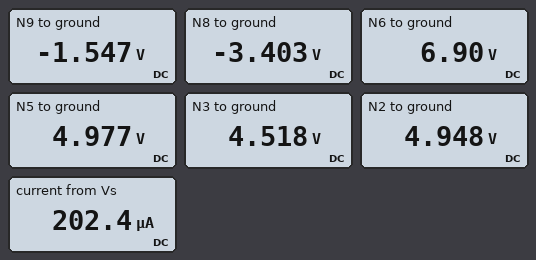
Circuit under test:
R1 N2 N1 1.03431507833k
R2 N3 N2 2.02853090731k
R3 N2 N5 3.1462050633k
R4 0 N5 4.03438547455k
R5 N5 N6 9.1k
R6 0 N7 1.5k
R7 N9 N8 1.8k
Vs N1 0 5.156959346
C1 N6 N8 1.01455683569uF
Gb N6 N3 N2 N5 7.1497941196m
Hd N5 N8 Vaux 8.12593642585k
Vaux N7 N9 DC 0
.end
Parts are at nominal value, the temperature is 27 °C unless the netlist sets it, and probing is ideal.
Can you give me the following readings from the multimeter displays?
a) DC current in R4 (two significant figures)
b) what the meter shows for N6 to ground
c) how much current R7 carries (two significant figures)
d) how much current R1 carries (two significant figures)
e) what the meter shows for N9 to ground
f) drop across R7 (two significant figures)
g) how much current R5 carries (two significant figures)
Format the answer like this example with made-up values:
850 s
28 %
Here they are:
1.2 mA
6.90 V
1.0 mA
200 µA
-1.547 V
1.9 V
210 µA
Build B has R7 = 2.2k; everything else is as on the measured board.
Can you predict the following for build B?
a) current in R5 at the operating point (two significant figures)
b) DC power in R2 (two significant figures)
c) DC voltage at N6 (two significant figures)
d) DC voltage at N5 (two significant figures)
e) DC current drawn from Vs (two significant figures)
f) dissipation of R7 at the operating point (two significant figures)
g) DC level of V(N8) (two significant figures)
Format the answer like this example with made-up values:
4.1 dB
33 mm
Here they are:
120 µA
27 µW
6.1 V
5.1 V
110 µA
2.9 mW
-4.2 V
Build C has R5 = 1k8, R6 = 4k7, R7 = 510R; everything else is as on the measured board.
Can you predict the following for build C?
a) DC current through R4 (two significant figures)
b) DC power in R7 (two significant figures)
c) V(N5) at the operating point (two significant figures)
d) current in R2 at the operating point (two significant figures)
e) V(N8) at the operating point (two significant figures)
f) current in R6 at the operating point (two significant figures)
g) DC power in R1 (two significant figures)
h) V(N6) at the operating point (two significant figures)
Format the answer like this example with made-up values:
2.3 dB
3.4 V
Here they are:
1.4 mA
1.9 mW
5.6 V
560 µA
-10 V
1.9 mA
300 µW
4.6 V
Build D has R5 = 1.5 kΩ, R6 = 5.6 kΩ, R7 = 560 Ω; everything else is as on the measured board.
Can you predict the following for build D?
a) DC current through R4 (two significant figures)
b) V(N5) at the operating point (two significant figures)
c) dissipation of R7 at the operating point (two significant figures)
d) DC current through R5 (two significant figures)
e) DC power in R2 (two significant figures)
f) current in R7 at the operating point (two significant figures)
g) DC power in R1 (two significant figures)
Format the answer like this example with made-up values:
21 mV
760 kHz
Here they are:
1.7 mA
6.7 V
6.5 mW
1.8 mA
6.8 mW
3.4 mA
3.2 mW
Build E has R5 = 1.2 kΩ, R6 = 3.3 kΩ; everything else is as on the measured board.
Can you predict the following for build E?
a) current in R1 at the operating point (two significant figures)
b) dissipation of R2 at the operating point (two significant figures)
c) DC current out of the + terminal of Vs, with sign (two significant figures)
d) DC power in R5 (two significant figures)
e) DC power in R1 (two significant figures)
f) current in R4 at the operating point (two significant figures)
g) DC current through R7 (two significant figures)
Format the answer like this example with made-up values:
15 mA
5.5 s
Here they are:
460 µA
470 µW
-460 µA
280 µW
220 µW
1.4 mA
1.8 mA
